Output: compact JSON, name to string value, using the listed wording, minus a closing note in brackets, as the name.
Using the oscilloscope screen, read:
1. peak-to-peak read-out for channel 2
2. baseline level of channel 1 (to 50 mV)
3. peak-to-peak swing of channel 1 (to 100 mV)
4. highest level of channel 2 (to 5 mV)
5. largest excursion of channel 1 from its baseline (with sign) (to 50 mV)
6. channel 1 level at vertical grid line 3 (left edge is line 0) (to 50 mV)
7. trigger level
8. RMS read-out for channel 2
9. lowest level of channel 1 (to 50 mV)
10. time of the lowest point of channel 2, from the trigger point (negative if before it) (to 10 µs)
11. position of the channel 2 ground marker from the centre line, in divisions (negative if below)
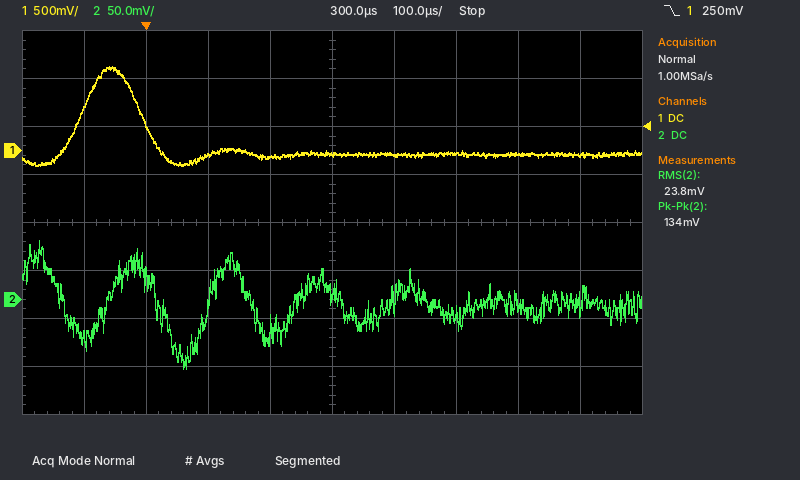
{"peak-to-peak read-out for channel 2": "134 mV", "baseline level of channel 1": "-50 mV", "peak-to-peak swing of channel 1": "1.00 V", "highest level of channel 2": "60 mV", "largest excursion of channel 1 from its baseline (with sign)": "+900 mV", "channel 1 level at vertical grid line 3 (left edge is line 0)": "-50 mV", "trigger level": "250 mV", "RMS read-out for channel 2": "23.8 mV", "lowest level of channel 1": "-150 mV", "time of the lowest point of channel 2, from the trigger point (negative if before it)": "+60 µs", "position of the channel 2 ground marker from the centre line, in divisions": "-1.6 div"}
